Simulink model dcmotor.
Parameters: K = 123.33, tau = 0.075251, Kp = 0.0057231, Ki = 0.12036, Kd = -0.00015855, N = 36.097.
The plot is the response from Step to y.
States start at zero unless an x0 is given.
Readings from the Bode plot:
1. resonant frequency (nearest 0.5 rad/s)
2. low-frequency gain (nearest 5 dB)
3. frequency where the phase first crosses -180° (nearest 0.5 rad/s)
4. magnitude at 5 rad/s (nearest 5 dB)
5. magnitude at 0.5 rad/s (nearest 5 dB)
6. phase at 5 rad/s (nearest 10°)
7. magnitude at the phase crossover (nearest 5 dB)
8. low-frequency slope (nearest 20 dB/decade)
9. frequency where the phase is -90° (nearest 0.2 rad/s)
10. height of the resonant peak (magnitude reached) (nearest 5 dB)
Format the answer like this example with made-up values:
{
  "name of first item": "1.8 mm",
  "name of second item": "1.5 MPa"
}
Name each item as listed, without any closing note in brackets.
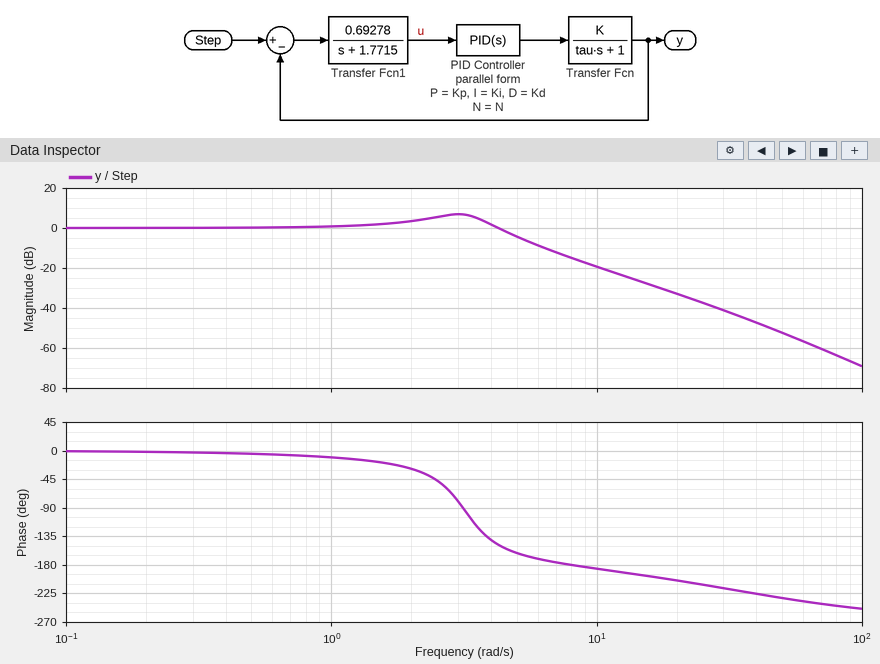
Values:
{
  "resonant frequency": "3.0 rad/s",
  "low-frequency gain": "0 dB",
  "frequency where the phase first crosses -180°": "8.0 rad/s",
  "magnitude at 5 rad/s": "-5 dB",
  "magnitude at 0.5 rad/s": "0 dB",
  "phase at 5 rad/s": "-160°",
  "magnitude at the phase crossover": "-15 dB",
  "low-frequency slope": "0 dB/decade",
  "frequency where the phase is -90°": "3.2 rad/s",
  "height of the resonant peak (magnitude reached)": "5 dB"
}
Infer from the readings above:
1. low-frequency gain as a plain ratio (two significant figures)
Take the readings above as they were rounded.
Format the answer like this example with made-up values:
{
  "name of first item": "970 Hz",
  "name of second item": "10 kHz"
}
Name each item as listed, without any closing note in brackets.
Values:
{
  "low-frequency gain as a plain ratio": "1.0"
}
